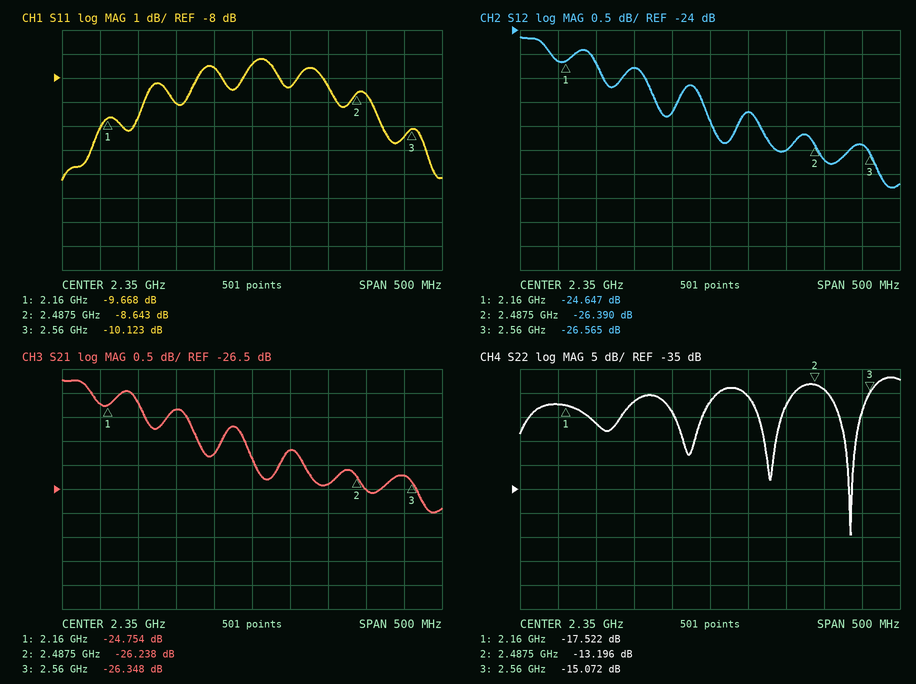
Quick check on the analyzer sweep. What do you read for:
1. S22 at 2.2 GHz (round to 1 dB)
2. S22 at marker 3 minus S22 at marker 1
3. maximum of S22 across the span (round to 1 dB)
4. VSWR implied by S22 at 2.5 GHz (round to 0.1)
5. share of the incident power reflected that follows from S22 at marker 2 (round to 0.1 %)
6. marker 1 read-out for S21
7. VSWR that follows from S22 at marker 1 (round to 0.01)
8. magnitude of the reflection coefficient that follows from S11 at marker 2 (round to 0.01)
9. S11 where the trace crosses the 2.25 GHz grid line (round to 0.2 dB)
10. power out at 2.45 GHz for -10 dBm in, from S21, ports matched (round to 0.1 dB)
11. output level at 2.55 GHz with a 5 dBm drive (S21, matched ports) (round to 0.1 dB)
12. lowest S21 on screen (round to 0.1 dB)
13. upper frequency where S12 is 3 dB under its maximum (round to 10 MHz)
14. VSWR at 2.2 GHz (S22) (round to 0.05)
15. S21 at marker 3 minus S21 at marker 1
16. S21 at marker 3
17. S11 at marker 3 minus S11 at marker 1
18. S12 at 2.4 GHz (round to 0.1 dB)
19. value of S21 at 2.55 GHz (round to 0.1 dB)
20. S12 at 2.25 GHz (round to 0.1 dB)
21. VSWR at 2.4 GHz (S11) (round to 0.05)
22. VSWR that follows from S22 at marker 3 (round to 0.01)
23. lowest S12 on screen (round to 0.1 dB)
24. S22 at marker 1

-21 dB
2.450 dB
-12 dB
1.5
4.8 %
-24.754 dB
1.31
0.37
-9.0 dB
-36.4 dBm
-21.2 dBm
-27.0 dB
2.58 GHz
1.20
-1.594 dB
-26.348 dB
-0.455 dB
-25.7 dB
-26.2 dB
-24.8 dB
2.25
1.43
-27.3 dB
-17.522 dB
